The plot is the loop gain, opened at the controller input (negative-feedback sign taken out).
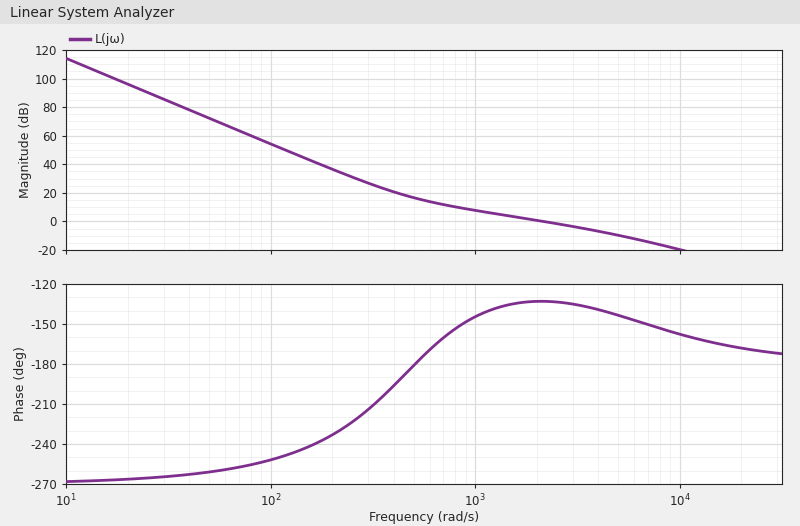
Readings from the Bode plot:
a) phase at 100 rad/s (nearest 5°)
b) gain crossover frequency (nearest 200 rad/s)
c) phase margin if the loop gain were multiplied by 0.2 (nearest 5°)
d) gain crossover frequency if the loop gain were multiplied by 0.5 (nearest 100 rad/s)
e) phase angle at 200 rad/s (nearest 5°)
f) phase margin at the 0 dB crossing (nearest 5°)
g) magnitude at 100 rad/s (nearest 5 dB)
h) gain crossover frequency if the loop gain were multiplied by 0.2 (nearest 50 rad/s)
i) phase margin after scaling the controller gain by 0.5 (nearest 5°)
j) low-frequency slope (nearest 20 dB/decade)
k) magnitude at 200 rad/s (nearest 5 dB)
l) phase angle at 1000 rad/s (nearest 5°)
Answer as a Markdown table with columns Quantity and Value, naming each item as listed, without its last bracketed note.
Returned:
| Quantity | Value |
|---|---|
| phase at 100 rad/s | -250° |
| gain crossover frequency | 2200 rad/s |
| phase margin if the loop gain were multiplied by 0.2 | 10° |
| gain crossover frequency if the loop gain were multiplied by 0.5 | 1200 rad/s |
| phase angle at 200 rad/s | -235° |
| phase margin at the 0 dB crossing | 45° |
| magnitude at 100 rad/s | 55 dB |
| gain crossover frequency if the loop gain were multiplied by 0.2 | 600 rad/s |
| phase margin after scaling the controller gain by 0.5 | 40° |
| low-frequency slope | -60 dB/decade |
| magnitude at 200 rad/s | 35 dB |
| phase angle at 1000 rad/s | -145° |
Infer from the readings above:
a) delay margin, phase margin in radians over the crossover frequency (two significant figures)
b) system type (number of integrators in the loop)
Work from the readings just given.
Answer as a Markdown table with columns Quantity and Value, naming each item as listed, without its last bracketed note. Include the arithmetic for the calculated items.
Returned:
| Quantity | Value |
|---|---|
| delay margin, phase margin in radians over the crossover frequency | 45 × π / 180 / 2200 = 0.00036 s |
| system type | 3 |
